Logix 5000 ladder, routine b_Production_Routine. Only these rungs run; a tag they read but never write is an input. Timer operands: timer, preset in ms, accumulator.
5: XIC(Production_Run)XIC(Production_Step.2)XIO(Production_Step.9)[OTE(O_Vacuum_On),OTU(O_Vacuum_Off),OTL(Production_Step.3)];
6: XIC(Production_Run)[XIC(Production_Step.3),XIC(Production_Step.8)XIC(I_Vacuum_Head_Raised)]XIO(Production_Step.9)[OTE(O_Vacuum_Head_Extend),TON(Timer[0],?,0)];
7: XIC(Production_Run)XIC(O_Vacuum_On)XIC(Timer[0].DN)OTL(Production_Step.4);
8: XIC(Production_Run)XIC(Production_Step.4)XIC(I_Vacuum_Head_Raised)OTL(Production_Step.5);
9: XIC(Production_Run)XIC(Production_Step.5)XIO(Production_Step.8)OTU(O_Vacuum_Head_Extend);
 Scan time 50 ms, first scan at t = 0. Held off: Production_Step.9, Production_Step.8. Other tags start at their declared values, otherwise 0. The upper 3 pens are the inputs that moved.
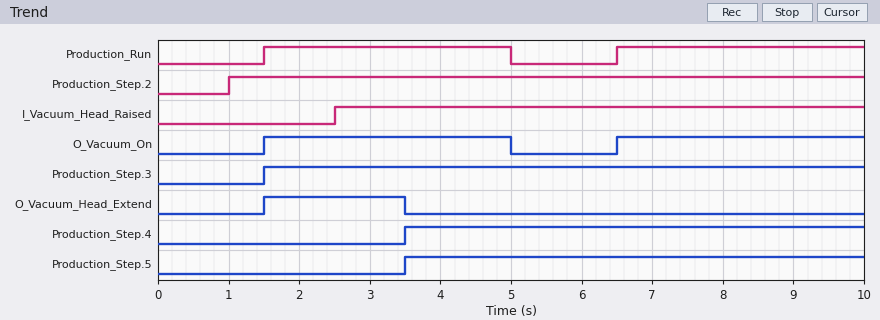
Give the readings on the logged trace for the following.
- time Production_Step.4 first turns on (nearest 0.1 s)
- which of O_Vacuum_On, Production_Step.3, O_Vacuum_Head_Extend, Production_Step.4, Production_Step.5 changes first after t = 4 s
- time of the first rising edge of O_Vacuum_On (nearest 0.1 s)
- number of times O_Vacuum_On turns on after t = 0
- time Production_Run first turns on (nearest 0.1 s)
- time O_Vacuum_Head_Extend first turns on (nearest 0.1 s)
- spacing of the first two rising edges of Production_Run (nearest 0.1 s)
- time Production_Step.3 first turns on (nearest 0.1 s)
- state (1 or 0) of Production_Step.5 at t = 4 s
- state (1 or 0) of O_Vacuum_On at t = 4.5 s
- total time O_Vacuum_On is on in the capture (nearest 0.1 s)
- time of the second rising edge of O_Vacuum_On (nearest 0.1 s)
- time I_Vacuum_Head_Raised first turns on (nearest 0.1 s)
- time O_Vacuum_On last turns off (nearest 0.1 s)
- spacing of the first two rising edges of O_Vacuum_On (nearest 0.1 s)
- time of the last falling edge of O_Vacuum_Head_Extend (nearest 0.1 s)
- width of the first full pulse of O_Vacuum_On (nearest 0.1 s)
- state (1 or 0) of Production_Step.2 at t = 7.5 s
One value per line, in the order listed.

3.5 s
O_Vacuum_On
1.5 s
2
1.5 s
1.5 s
5.0 s
1.5 s
1
1
7.0 s
6.5 s
2.5 s
5.0 s
5.0 s
3.5 s
3.5 s
1
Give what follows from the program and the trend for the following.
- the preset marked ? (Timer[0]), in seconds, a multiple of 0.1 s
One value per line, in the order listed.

2.0 s
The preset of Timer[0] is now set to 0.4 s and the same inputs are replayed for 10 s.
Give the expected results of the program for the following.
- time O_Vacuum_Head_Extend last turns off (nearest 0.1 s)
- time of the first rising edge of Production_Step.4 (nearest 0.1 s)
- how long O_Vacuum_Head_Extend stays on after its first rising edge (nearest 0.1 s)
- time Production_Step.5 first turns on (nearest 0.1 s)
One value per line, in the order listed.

2.5 s
1.9 s
1.0 s
2.5 s
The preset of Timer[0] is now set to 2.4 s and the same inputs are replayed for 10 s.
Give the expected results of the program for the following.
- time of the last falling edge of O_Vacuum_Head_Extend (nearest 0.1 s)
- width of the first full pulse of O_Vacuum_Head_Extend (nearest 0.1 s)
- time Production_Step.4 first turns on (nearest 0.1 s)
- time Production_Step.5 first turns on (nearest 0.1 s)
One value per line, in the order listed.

3.9 s
2.4 s
3.9 s
3.9 s
